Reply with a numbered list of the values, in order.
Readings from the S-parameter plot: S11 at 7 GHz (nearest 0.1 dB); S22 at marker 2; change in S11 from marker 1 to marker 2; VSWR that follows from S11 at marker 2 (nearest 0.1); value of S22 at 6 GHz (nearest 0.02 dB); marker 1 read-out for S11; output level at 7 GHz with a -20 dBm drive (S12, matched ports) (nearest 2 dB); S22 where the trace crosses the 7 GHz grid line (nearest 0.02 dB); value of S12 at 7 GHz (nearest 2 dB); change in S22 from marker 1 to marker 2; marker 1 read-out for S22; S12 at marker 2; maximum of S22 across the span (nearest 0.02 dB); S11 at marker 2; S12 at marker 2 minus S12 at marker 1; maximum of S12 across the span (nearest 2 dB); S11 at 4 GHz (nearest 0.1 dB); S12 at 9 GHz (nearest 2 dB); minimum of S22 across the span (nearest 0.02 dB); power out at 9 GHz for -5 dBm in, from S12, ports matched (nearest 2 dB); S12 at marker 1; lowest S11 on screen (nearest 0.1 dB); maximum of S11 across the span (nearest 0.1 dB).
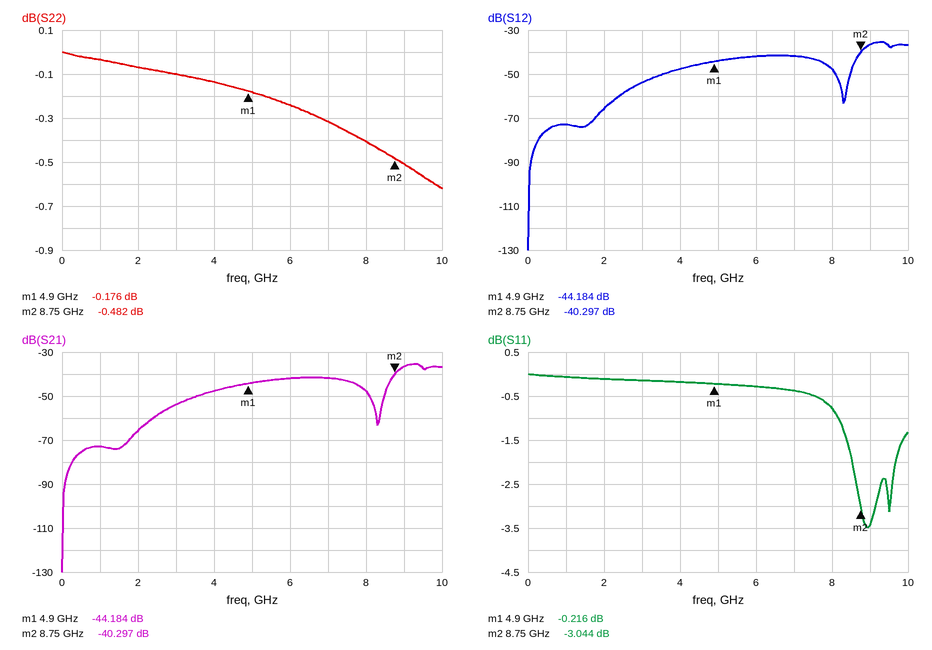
1. -0.4 dB
2. -0.482 dB
3. -2.828 dB
4. 5.8
5. -0.24 dB
6. -0.216 dB
7. -62 dBm
8. -0.32 dB
9. -42 dB
10. -0.306 dB
11. -0.176 dB
12. -40.297 dB
13. 0.00 dB
14. -3.044 dB
15. 3.887 dB
16. -36 dB
17. -0.2 dB
18. -36 dB
19. -0.62 dB
20. -42 dBm
21. -44.184 dB
22. -3.5 dB
23. 0.0 dB
